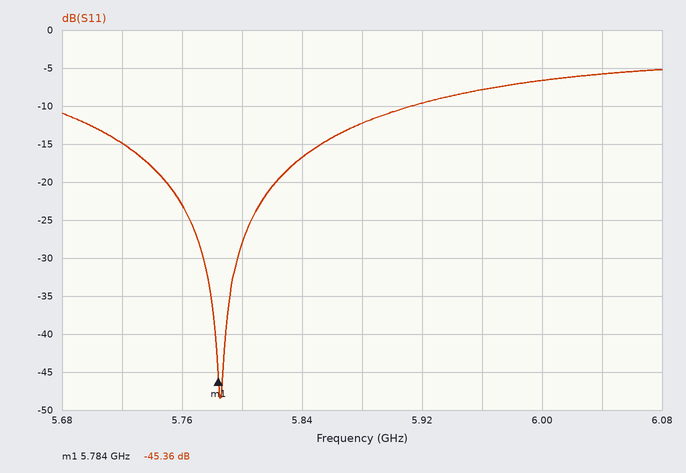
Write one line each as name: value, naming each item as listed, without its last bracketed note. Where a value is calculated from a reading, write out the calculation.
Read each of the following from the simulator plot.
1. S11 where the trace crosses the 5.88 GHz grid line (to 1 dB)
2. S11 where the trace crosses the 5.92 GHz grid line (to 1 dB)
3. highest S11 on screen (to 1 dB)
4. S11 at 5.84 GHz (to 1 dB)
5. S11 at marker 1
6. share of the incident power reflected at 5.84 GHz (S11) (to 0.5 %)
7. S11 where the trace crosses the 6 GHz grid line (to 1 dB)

S11 where the trace crosses the 5.88 GHz grid line: -12 dB
S11 where the trace crosses the 5.92 GHz grid line: -10 dB
highest S11 on screen: -5 dB
S11 at 5.84 GHz: -17 dB
S11 at marker 1: -45.36 dB
share of the incident power reflected at 5.84 GHz (S11): 10^(-17/10) ≈ 2.0 %
S11 where the trace crosses the 6 GHz grid line: -7 dB
